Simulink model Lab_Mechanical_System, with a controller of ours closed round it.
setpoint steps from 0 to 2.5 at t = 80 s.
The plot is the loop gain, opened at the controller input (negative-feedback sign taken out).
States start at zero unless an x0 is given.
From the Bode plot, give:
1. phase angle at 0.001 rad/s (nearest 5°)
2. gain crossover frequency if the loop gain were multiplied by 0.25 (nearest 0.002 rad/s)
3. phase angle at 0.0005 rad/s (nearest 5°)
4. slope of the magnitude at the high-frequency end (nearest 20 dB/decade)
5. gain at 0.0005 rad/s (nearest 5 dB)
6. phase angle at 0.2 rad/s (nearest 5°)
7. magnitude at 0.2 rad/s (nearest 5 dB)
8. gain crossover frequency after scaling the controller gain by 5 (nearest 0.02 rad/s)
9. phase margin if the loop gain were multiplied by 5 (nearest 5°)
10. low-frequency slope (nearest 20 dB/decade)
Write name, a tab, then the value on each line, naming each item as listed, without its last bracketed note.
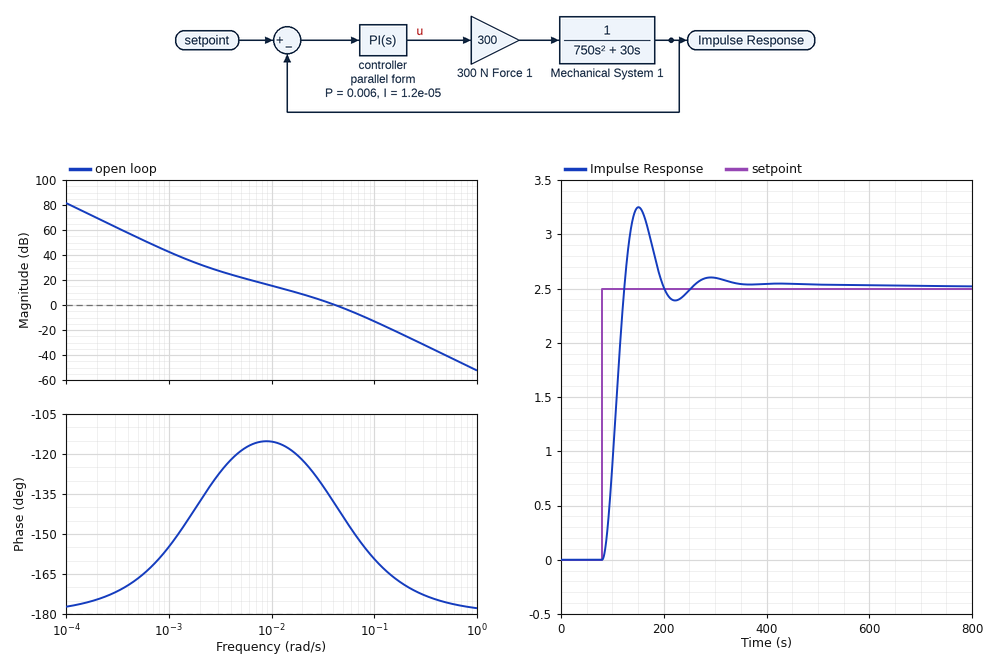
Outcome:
phase angle at 0.001 rad/s	-155°
gain crossover frequency if the loop gain were multiplied by 0.25	0.014 rad/s
phase angle at 0.0005 rad/s	-165°
slope of the magnitude at the high-frequency end	-40 dB/decade
gain at 0.0005 rad/s	55 dB
phase angle at 0.2 rad/s	-170°
magnitude at 0.2 rad/s	-25 dB
gain crossover frequency after scaling the controller gain by 5	0.10 rad/s
phase margin if the loop gain were multiplied by 5	20°
low-frequency slope	-40 dB/decade
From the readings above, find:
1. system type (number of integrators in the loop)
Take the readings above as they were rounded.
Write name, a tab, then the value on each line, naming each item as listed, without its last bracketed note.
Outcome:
system type	2
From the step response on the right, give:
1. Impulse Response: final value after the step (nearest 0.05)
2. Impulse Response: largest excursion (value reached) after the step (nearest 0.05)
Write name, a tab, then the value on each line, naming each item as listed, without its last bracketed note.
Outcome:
Impulse Response: final value after the step	2.50
Impulse Response: largest excursion (value reached) after the step	3.25
